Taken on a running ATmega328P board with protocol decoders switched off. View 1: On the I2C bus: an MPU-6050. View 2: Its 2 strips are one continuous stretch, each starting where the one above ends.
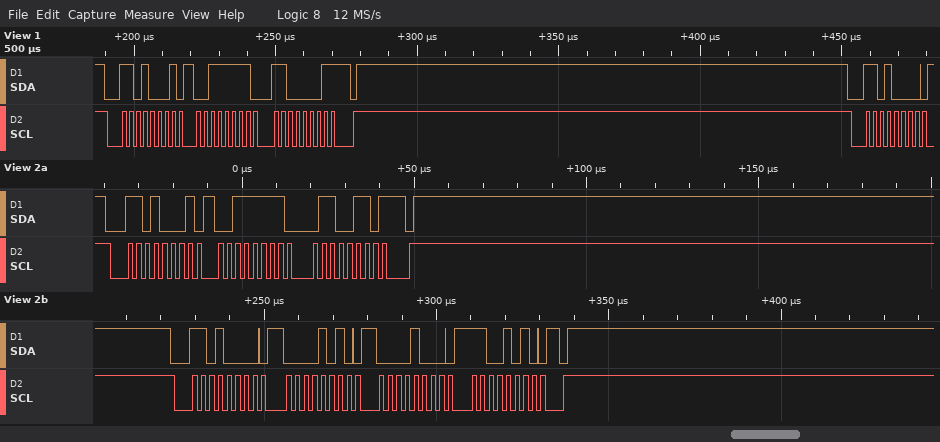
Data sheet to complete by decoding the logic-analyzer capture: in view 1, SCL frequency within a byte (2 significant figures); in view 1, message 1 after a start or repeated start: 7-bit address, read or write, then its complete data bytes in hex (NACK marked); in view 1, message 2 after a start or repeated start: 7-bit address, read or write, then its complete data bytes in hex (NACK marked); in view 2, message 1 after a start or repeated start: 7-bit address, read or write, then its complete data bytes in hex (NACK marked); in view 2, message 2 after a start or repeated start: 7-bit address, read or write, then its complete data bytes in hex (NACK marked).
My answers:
400 kHz
0x68 read: 3F C1 NACK
0x68 write
0x68 read: 3F 66 NACK
0x68 write: 0A 08 CA
